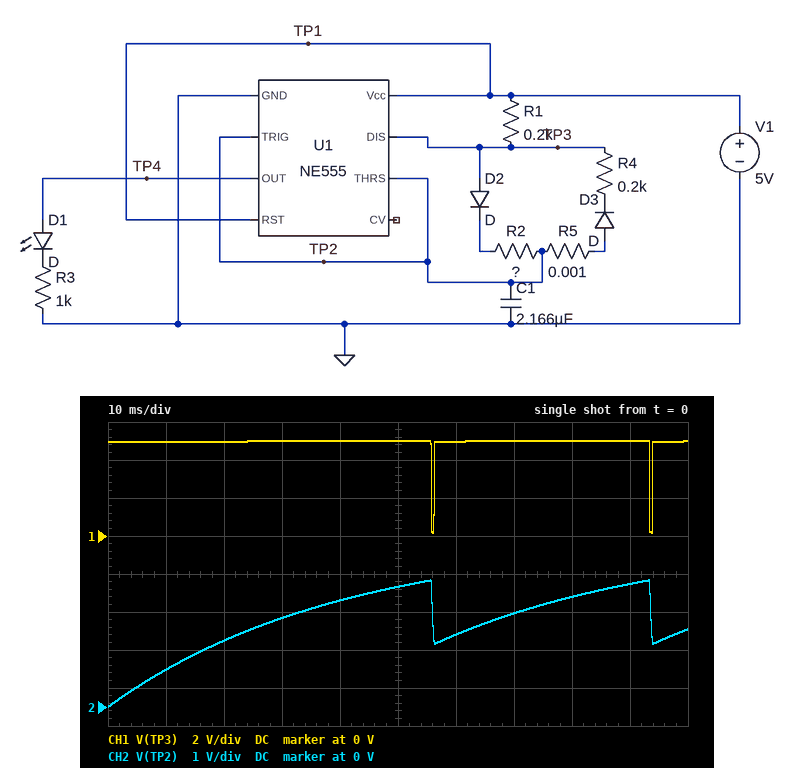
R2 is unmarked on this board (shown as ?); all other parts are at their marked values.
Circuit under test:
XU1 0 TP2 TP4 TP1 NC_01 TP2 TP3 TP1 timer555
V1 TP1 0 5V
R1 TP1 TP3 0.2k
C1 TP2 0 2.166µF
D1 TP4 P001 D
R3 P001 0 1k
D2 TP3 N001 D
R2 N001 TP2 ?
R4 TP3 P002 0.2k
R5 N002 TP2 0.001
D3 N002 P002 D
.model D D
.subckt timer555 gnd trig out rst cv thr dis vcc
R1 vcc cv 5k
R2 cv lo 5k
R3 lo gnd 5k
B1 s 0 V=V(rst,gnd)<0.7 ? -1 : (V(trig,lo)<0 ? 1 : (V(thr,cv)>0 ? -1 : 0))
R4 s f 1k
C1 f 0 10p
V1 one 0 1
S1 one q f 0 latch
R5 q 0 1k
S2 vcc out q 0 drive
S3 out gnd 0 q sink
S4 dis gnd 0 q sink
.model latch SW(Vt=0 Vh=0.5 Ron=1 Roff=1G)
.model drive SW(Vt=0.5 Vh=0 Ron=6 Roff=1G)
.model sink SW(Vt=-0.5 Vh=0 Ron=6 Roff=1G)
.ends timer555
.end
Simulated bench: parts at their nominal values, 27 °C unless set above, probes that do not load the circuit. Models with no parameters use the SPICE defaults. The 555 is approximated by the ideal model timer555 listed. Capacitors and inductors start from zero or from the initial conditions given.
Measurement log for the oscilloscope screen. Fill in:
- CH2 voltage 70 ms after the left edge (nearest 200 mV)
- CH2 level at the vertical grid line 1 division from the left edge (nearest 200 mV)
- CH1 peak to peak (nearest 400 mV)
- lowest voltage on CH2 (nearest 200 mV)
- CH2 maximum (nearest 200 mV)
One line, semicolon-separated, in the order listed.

2.4 V; 1.0 V; 4.8 V; 0 V; 3.4 V
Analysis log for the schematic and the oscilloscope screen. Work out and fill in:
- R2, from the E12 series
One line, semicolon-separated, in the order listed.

18 kΩ
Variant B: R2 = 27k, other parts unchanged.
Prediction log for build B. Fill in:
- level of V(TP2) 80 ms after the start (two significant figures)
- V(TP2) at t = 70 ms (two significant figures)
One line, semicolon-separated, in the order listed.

3.3 V; 3.1 V
